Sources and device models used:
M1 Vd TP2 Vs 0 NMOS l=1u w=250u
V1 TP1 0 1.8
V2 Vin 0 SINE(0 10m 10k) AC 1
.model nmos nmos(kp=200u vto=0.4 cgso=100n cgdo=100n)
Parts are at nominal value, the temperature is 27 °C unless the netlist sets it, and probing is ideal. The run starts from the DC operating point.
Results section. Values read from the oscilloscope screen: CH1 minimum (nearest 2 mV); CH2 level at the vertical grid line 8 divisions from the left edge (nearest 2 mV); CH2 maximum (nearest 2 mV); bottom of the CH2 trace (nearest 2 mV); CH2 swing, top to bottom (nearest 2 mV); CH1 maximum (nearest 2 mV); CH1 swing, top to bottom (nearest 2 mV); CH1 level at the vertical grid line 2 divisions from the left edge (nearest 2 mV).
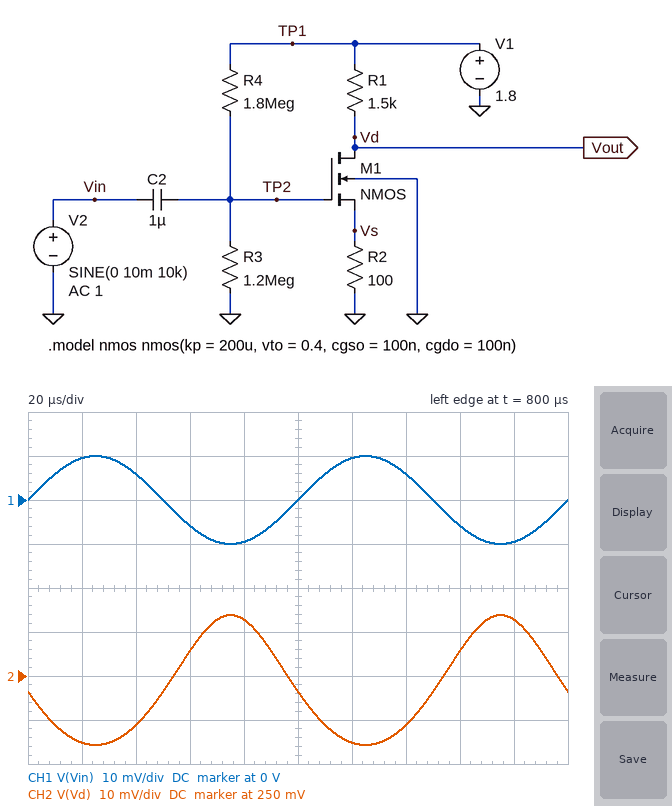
-10 mV
256 mV
264 mV
234 mV
30 mV
10 mV
20 mV
6 mV
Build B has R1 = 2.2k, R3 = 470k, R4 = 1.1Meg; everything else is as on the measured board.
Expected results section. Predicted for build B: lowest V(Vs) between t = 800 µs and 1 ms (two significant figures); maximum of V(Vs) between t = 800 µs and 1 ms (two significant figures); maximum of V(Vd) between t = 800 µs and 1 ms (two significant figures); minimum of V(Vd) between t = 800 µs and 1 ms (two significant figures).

26 mV
33 mV
1.2 V
1.1 V
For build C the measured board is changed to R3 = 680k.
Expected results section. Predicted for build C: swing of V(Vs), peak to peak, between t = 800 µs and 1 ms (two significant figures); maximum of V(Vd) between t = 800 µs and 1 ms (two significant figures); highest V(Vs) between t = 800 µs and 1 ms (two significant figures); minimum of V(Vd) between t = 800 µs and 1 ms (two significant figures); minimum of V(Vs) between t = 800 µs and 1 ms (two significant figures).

5.6 mV
1.6 V
18 mV
1.5 V
13 mV
